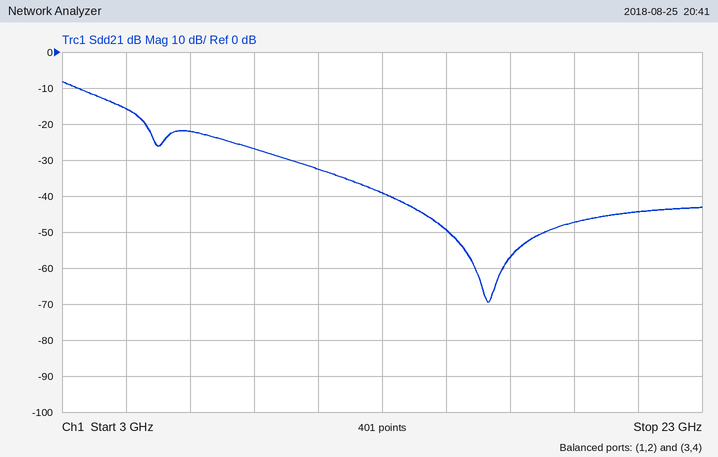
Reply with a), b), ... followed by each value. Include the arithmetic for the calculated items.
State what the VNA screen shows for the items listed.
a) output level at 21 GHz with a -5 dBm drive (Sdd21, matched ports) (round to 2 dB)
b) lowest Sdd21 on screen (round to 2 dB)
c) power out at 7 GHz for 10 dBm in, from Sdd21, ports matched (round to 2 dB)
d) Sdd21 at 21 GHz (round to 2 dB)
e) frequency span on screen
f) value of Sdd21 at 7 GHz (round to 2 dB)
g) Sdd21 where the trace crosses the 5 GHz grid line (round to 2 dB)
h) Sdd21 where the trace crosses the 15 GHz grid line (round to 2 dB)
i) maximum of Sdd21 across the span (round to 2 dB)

a) -5 dBm + (-44 dB) = -50 dBm
b) -70 dB
c) 10 dBm + (-22 dB) = -12 dBm
d) -44 dB
e) 20 GHz
f) -22 dB
g) -16 dB
h) -50 dB
i) -8 dB
